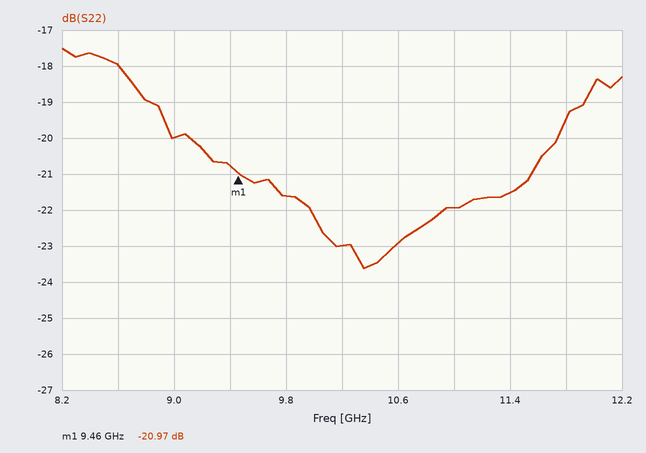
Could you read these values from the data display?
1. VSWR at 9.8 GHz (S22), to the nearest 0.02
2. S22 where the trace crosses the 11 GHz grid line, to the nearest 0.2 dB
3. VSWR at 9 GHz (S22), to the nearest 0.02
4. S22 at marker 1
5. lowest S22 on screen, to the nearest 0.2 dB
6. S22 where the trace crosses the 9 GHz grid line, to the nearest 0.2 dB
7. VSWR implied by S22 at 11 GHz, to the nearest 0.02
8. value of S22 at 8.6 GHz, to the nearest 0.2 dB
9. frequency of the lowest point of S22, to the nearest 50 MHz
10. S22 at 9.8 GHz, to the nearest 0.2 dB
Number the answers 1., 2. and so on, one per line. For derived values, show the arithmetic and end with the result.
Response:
1. |Γ| = 10^(-21.6/20) = 0.0832; VSWR = (1 + 0.0832)/(1 − 0.0832) ≈ 1.18
2. -22.0 dB
3. |Γ| = 10^(-20/20) = 0.1000; VSWR = (1 + 0.1000)/(1 − 0.1000) ≈ 1.22
4. -20.97 dB
5. -23.6 dB
6. -20.0 dB
7. |Γ| = 10^(-22/20) = 0.0794; VSWR = (1 + 0.0794)/(1 − 0.0794) ≈ 1.17, so 1.18 to the nearest 0.02
8. -18.0 dB
9. 10.35 GHz
10. -21.6 dB
